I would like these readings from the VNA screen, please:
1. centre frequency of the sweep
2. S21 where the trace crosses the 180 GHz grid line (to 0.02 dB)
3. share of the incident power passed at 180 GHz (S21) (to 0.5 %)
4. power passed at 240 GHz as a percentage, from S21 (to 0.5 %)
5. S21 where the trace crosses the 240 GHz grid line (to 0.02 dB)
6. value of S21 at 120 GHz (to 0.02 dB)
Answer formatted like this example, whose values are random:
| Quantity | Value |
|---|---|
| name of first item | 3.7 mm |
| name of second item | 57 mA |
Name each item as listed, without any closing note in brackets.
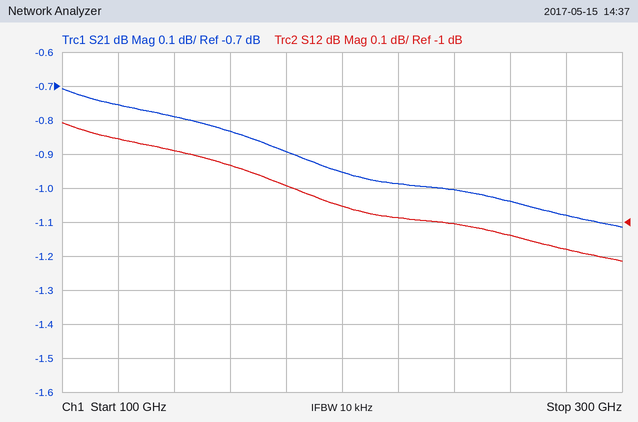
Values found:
| Quantity | Value |
|---|---|
| centre frequency of the sweep | 200 GHz |
| S21 where the trace crosses the 180 GHz grid line | -0.90 dB |
| share of the incident power passed at 180 GHz (S21) | 81.5 % |
| power passed at 240 GHz as a percentage, from S21 | 79.5 % |
| S21 where the trace crosses the 240 GHz grid line | -1.00 dB |
| value of S21 at 120 GHz | -0.76 dB |
